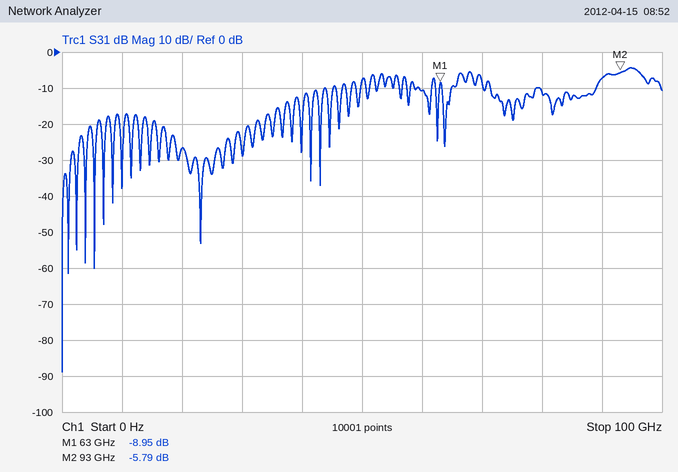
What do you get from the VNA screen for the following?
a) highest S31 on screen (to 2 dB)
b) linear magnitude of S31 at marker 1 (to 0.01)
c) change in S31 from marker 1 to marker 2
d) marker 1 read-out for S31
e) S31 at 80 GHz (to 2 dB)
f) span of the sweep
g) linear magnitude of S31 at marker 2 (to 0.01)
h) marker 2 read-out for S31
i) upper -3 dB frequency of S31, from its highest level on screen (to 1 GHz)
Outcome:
-4 dB
0.36
3.16 dB
-8.95 dB
-12 dB
100 GHz
0.51
-5.79 dB
97 GHz
